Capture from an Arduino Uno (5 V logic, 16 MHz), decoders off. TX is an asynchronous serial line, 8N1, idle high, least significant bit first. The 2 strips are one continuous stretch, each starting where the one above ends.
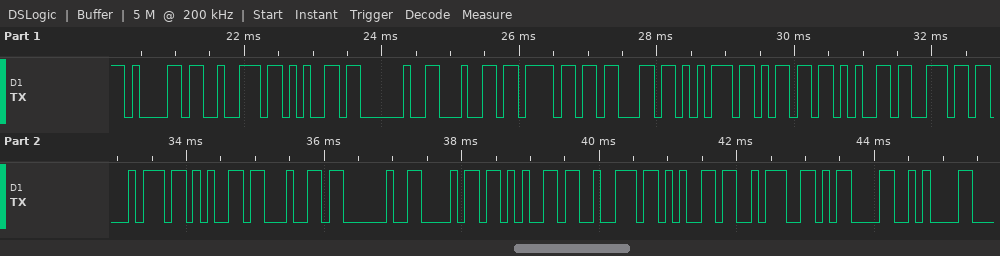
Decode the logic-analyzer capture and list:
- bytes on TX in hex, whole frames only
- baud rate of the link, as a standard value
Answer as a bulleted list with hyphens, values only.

- 61 72 65 20 64 6F 63 75 6D 65 6E 74 65 64 20 68 65 72 65 3A 0D 0A
- 9600 baud
